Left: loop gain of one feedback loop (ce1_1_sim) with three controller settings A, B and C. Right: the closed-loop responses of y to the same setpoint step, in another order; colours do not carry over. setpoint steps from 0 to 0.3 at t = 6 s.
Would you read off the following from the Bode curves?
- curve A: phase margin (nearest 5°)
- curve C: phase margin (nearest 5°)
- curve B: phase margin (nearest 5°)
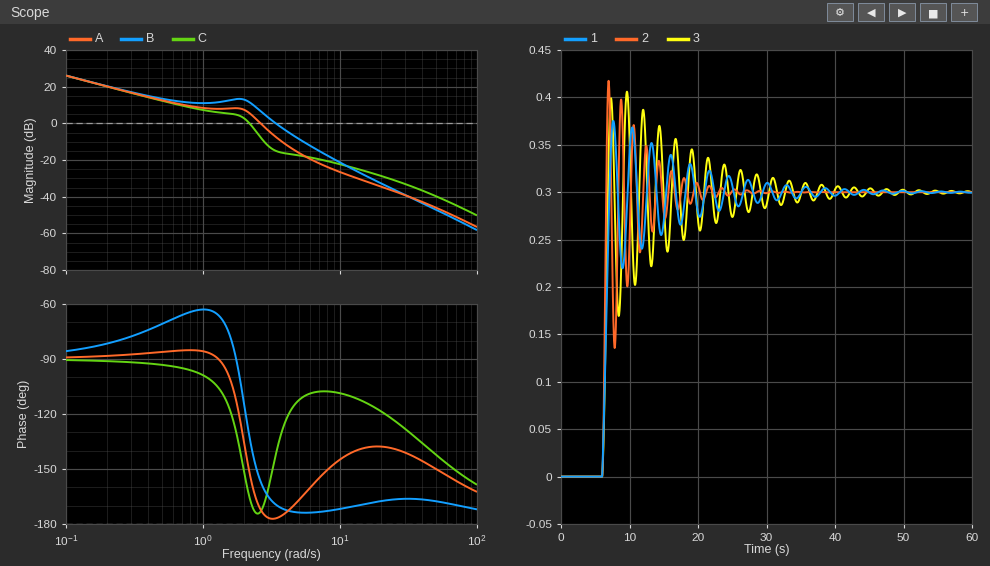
10°
15°
10°
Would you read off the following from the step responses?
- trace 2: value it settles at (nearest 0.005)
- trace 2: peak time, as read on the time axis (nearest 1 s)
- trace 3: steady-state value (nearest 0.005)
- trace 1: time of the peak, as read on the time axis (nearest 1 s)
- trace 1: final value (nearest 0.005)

0.300
7 s
0.300
8 s
0.300
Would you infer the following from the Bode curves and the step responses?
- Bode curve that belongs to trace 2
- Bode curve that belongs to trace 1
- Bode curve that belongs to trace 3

B
C
A
